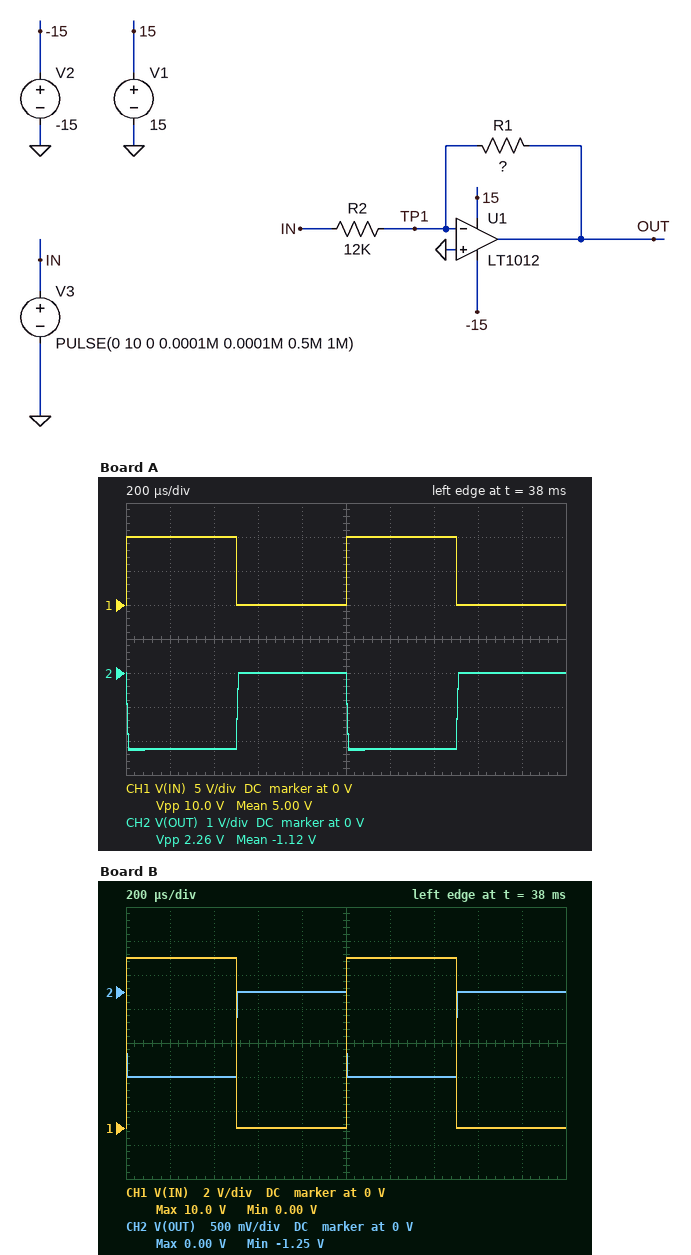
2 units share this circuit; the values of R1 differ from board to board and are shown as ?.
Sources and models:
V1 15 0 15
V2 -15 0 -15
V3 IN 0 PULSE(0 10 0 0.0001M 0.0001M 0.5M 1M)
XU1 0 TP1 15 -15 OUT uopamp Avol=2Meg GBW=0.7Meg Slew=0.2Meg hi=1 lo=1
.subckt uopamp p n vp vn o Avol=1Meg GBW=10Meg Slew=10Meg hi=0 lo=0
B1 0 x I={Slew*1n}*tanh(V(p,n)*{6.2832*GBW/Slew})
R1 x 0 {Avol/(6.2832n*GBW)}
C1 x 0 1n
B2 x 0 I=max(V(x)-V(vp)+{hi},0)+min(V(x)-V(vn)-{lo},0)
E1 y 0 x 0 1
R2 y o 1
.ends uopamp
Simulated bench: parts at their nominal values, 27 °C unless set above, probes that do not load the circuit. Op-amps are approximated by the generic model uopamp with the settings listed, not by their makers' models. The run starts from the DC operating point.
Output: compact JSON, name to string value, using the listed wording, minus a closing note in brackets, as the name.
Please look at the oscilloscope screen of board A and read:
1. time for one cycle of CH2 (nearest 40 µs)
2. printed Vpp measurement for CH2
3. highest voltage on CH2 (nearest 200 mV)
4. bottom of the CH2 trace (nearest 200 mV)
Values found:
{"time for one cycle of CH2": "1.00 ms", "printed Vpp measurement for CH2": "2.26 V", "highest voltage on CH2": "0 V", "bottom of the CH2 trace": "-2.2 V"}
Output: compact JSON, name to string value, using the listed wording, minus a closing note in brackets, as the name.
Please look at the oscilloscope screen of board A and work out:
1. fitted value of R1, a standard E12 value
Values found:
{"fitted value of R1, a standard E12 value": "2.7 kΩ"}
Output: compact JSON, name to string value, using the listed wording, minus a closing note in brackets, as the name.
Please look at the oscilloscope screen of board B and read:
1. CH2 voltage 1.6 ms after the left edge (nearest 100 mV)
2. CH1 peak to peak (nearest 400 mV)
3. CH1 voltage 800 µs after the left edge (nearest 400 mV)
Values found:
{"CH2 voltage 1.6 ms after the left edge": "0 V", "CH1 peak to peak": "10.0 V", "CH1 voltage 800 µs after the left edge": "0 V"}
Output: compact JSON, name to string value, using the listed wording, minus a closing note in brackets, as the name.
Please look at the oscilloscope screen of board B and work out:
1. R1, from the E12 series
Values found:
{"R1, from the E12 series": "1.5 kΩ"}
